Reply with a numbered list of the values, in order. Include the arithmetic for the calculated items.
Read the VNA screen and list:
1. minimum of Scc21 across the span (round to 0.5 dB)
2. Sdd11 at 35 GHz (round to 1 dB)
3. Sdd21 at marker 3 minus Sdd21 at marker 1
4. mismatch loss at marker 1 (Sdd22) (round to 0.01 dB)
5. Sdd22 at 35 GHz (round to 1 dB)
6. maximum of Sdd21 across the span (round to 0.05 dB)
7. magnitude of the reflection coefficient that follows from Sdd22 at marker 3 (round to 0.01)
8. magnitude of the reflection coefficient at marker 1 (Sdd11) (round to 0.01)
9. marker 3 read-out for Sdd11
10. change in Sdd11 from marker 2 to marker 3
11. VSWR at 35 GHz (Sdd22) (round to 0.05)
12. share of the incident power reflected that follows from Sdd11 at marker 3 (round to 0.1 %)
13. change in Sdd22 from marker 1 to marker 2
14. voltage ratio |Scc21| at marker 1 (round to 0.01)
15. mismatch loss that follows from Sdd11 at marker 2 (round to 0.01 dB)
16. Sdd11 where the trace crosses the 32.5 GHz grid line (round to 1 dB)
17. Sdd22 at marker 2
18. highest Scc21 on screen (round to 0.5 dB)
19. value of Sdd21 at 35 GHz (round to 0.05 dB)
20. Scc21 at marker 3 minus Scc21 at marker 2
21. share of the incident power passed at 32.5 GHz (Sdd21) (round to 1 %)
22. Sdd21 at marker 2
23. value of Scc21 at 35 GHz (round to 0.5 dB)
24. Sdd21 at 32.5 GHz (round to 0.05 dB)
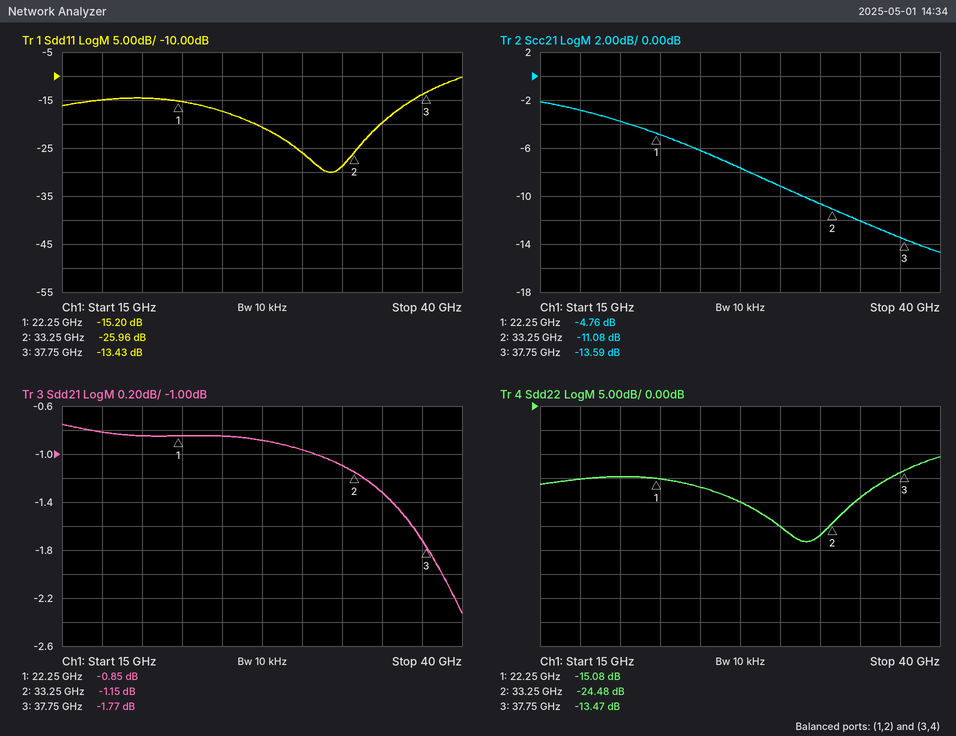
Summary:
1. -14.5 dB
2. -20 dB
3. -1.77 − (-0.85) = -0.92 dB
4. −10 log10(1 − 10^(-15.08/10)) ≈ 0.14 dB
5. -19 dB
6. -0.75 dB
7. 10^(-13.47/20) ≈ 0.21
8. 10^(-15.2/20) ≈ 0.17
9. -13.43 dB
10. -13.43 − (-25.96) = 12.53 dB
11. |Γ| = 10^(-19/20) = 0.1122; VSWR = (1 + 0.1122)/(1 − 0.1122) ≈ 1.25
12. 10^(-13.43/10) ≈ 4.5 %
13. -24.48 − (-15.08) = -9.40 dB
14. 10^(-4.76/20) ≈ 0.58
15. −10 log10(1 − 10^(-25.96/10)) ≈ 0.01 dB
16. -29 dB
17. -24.48 dB
18. -2.0 dB
19. -1.30 dB
20. -13.59 − (-11.08) = -2.51 dB
21. 10^(-1.1/10) ≈ 78 %
22. -1.15 dB
23. -12.0 dB
24. -1.10 dB
